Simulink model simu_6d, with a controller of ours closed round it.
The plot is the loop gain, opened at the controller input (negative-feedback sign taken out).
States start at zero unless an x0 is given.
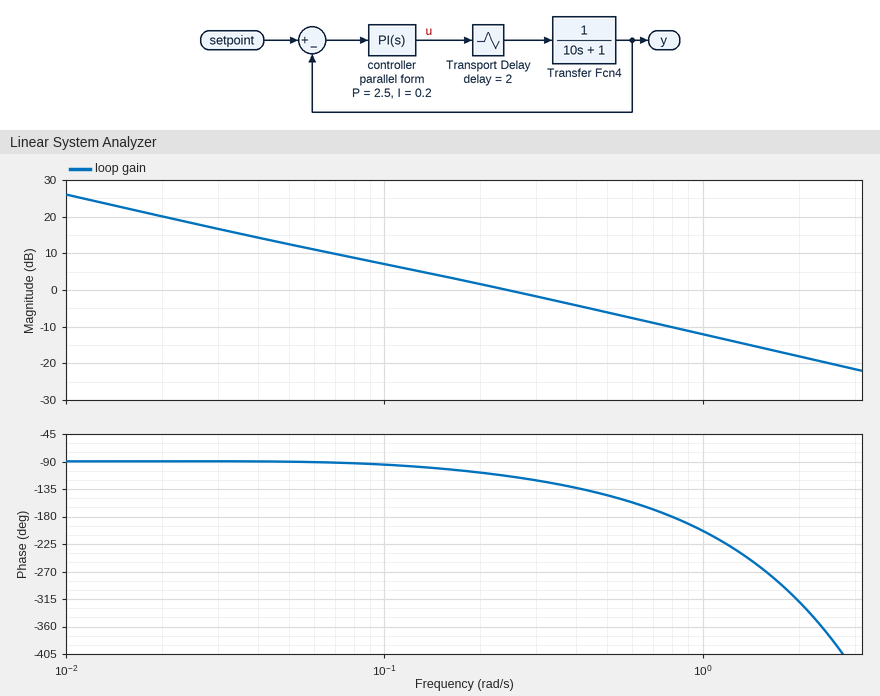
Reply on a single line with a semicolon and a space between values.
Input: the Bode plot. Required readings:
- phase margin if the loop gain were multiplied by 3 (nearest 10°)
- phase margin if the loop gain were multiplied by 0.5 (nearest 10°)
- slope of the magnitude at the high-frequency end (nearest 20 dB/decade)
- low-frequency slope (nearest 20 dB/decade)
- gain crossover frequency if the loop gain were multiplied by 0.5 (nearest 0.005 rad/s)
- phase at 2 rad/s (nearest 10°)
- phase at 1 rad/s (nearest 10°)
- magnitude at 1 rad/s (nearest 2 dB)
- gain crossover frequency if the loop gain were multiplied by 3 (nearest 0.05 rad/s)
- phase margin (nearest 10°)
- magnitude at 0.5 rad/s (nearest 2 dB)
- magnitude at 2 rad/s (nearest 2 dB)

10°; 80°; -20 dB/decade; -20 dB/decade; 0.115 rad/s; -320°; -200°; -12 dB; 0.75 rad/s; 70°; -6 dB; -18 dB
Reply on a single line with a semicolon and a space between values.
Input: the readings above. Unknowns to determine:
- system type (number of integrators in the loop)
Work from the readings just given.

1
